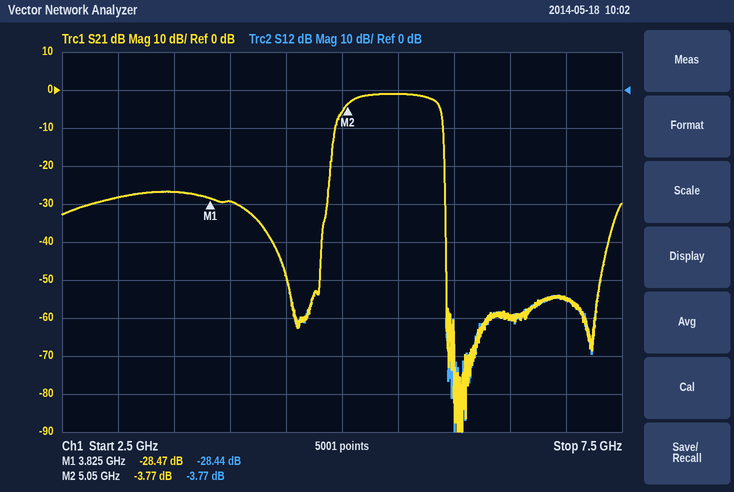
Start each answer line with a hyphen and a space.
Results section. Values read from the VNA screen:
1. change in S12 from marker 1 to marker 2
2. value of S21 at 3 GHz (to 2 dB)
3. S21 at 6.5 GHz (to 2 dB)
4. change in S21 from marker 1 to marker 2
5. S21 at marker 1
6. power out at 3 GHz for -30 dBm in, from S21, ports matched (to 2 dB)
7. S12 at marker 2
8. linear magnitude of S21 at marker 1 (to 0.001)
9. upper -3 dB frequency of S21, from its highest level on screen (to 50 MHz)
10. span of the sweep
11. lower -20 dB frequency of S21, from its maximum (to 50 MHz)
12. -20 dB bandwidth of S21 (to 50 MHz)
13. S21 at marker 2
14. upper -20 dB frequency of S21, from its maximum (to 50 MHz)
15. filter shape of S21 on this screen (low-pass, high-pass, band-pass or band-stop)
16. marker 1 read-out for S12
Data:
- 24.67 dB
- -28 dB
- -60 dB
- 24.70 dB
- -28.47 dB
- -58 dBm
- -3.77 dB
- 0.038
- 5.85 GHz
- 5 GHz
- 4.90 GHz
- 1.00 GHz
- -3.77 dB
- 5.90 GHz
- band-pass
- -28.44 dB
